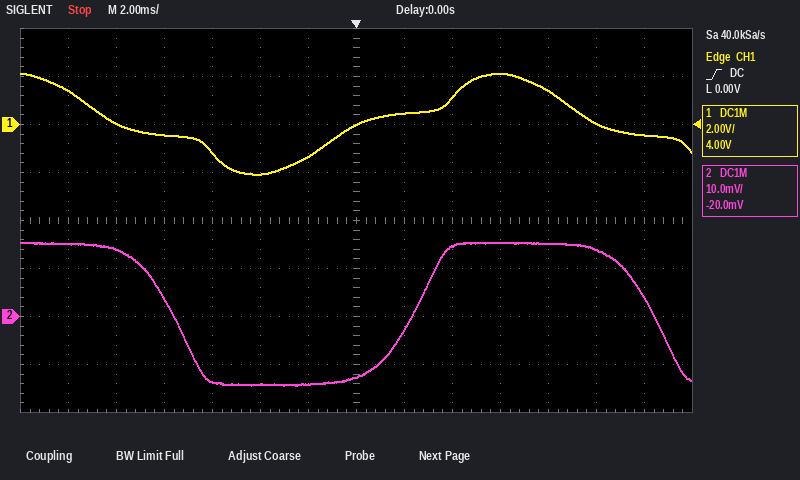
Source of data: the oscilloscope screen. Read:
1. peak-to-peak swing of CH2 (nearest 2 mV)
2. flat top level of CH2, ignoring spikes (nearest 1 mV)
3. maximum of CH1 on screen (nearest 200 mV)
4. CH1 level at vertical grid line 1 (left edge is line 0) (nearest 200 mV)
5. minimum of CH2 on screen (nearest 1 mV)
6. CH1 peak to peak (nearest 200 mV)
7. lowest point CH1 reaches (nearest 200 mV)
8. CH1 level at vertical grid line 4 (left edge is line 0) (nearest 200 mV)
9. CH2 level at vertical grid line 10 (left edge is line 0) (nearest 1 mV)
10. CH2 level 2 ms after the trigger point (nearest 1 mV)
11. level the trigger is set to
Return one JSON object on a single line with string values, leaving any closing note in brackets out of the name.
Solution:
{"peak-to-peak swing of CH2": "30 mV", "flat top level of CH2, ignoring spikes": "15 mV", "maximum of CH1 on screen": "2.2 V", "CH1 level at vertical grid line 1 (left edge is line 0)": "1.4 V", "minimum of CH2 on screen": "-14 mV", "CH1 peak to peak": "4.2 V", "lowest point CH1 reaches": "-2.0 V", "CH1 level at vertical grid line 4 (left edge is line 0)": "-1.2 V", "CH2 level at vertical grid line 10 (left edge is line 0)": "15 mV", "CH2 level 2 ms after the trigger point": "-3 mV", "level the trigger is set to": "0.00 V"}
